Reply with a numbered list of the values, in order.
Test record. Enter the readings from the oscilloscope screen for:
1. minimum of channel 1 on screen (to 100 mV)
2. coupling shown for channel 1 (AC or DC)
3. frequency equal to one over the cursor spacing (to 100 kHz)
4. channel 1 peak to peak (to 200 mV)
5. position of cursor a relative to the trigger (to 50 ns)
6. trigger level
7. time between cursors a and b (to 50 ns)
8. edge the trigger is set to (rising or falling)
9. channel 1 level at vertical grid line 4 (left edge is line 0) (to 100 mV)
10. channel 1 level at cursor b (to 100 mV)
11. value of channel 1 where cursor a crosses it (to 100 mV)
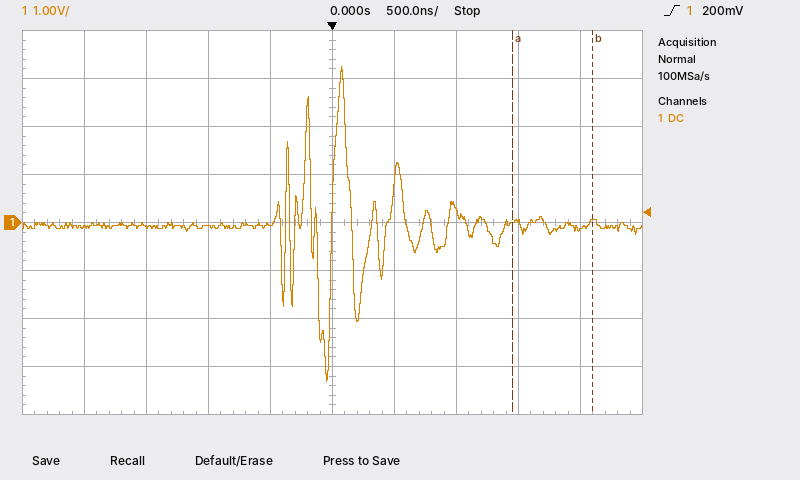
1. -3.3 V
2. DC
3. 1.5 MHz
4. 6.6 V
5. +1.45 µs
6. 200 mV
7. 650 ns
8. rising
9. 0.0 V
10. 0.0 V
11. 0.0 V
